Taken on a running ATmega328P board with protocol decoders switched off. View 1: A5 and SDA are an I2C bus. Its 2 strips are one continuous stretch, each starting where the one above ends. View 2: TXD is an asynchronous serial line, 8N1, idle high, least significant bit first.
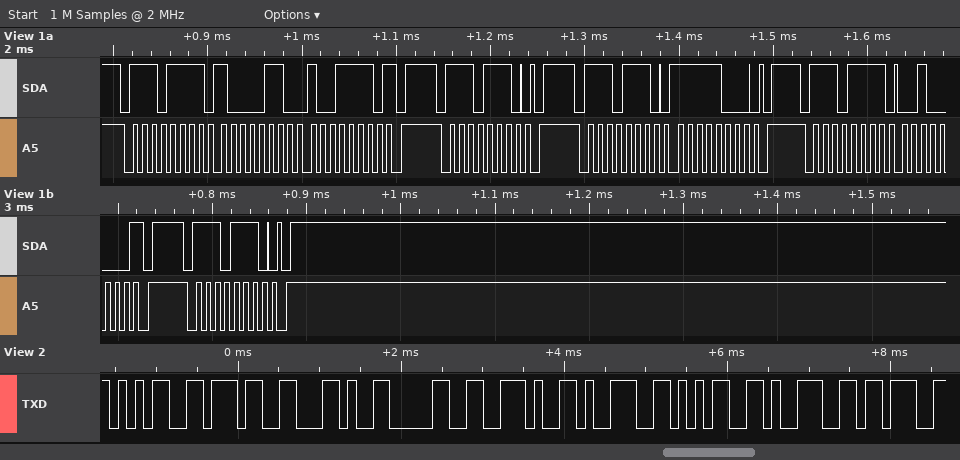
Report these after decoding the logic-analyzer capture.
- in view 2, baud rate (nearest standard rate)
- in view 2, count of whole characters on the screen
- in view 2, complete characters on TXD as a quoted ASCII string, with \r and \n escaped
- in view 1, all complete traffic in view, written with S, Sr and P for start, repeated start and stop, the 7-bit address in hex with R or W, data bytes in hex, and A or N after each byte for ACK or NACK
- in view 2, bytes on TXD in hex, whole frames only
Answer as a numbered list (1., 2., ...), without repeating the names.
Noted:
1. 9600 baud
2. 9
3. "57,0.959;"
4. S 77R A 86 A 9E N P S 77W A P S 77W A F8 A P S 77R A 20 N P S 77W A P
5. 35 37 2C 30 2E 39 35 39 3B
